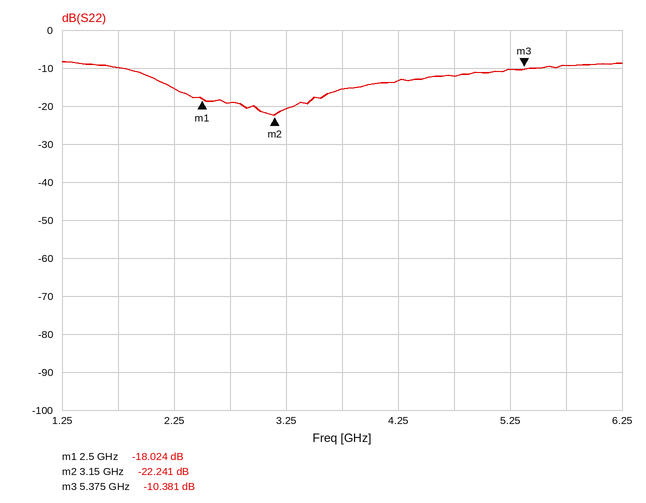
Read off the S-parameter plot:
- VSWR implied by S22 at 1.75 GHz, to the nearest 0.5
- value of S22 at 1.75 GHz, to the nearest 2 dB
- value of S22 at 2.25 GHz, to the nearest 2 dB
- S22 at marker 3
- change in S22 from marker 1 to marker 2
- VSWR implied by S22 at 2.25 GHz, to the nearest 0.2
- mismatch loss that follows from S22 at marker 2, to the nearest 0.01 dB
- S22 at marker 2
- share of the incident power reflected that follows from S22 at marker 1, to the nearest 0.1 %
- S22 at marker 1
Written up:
2.0
-10 dB
-16 dB
-10.381 dB
-4.217 dB
1.4
0.03 dB
-22.241 dB
1.6 %
-18.024 dB
